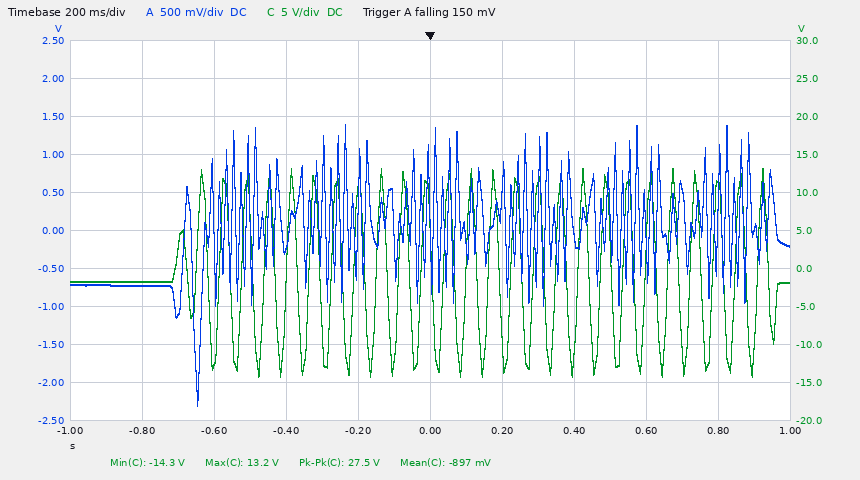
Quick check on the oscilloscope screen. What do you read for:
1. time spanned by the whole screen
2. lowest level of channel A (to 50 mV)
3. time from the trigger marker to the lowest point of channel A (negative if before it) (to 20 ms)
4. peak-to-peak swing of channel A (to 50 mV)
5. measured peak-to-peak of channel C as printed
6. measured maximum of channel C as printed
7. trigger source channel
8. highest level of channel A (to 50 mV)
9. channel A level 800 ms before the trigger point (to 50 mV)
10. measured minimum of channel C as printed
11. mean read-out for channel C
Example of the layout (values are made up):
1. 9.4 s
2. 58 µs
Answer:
1. 2 s
2. -2.30 V
3. -640 ms
4. 3.70 V
5. 27.5 V
6. 13.2 V
7. channel A
8. 1.40 V
9. -700 mV
10. -14.3 V
11. -897 mV
